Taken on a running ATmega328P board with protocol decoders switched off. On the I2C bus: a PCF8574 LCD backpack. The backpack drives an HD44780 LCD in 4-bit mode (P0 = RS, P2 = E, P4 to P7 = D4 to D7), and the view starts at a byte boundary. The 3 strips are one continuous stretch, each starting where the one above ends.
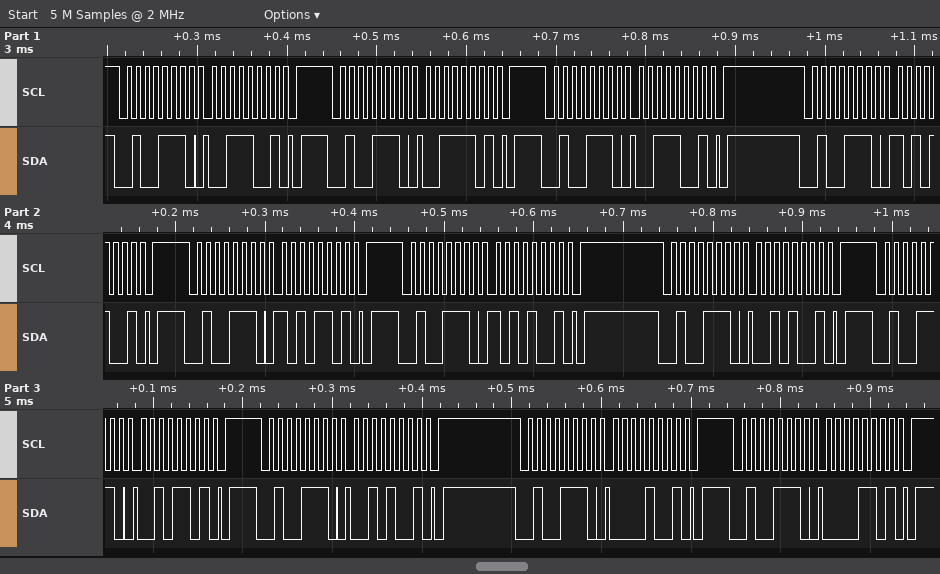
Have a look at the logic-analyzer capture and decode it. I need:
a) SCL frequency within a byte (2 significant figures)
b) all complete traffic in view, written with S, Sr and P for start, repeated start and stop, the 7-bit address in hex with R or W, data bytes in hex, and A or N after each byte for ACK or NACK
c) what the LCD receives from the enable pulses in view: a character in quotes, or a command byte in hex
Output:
100 kHz
S 27W A 39 A P S 27W A 3D A P S 27W A 39 A P S 27W A A9 A P S 27W A AD A P S 27W A A9 A P S 27W A 29 A P S 27W A 2D A P S 27W A 29 A P S 27W A 09 A P S 27W A 0D A P
':'
